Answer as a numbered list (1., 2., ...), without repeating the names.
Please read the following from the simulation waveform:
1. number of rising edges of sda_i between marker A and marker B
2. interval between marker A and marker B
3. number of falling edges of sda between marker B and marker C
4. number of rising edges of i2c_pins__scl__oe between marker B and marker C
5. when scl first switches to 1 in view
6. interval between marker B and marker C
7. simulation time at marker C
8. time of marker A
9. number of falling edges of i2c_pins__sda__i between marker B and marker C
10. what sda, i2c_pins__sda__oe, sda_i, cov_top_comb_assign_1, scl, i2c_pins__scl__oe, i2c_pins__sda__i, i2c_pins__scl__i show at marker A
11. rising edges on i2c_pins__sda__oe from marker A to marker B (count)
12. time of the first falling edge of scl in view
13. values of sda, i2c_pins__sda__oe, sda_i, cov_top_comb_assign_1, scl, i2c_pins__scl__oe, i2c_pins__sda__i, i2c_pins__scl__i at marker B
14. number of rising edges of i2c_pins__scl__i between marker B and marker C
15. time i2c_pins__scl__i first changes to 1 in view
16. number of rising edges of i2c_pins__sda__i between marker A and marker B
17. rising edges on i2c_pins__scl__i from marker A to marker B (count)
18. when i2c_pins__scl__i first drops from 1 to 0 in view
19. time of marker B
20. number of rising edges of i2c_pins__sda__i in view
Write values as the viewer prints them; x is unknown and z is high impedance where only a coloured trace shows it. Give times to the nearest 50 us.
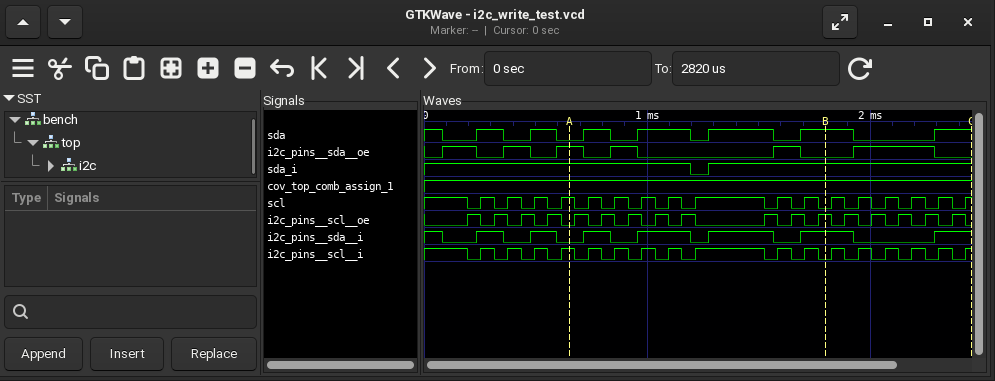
1. 1
2. 1150 us
3. 1
4. 5
5. 250 us
6. 650 us
7. 2450 us
8. 650 us
9. 1
10. sda=0, i2c_pins__sda__oe=1, sda_i=1, cov_top_comb_assign_1=1, scl=1, i2c_pins__scl__oe=0, i2c_pins__sda__i=0, i2c_pins__scl__i=1
11. 2
12. 200 us
13. sda=1, i2c_pins__sda__oe=0, sda_i=1, cov_top_comb_assign_1=1, scl=0, i2c_pins__scl__oe=1, i2c_pins__sda__i=1, i2c_pins__scl__i=0
14. 6
15. 250 us
16. 4
17. 7
18. 200 us
19. 1800 us
20. 7
